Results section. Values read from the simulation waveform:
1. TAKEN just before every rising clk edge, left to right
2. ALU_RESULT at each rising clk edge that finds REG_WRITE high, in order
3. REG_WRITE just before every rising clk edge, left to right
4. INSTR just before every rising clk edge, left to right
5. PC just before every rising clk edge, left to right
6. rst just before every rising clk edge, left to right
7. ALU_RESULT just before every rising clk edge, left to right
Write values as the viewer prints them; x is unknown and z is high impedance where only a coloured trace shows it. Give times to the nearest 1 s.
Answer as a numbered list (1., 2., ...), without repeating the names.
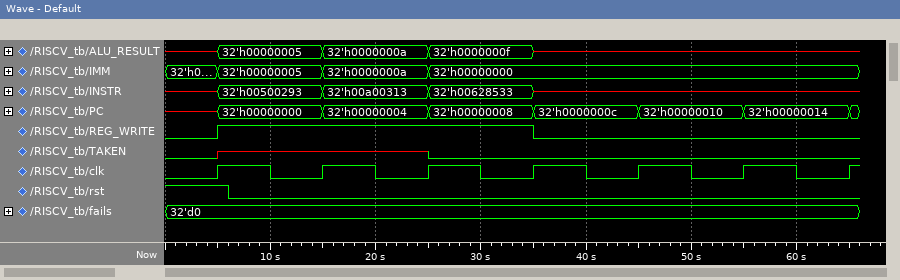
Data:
1. 0 x x 0 0 0 0
2. 32'h00000005, 32'h0000000a, 32'h0000000f
3. 0 1 1 1 0 0 0
4. x, 32'h00500293, 32'h00a00313, 32'h00628533, x, x, x
5. x, 32'h00000000, 32'h00000004, 32'h00000008, 32'h0000000c, 32'h00000010, 32'h00000014
6. 1 0 0 0 0 0 0
7. x, 32'h00000005, 32'h0000000a, 32'h0000000f, x, x, x
